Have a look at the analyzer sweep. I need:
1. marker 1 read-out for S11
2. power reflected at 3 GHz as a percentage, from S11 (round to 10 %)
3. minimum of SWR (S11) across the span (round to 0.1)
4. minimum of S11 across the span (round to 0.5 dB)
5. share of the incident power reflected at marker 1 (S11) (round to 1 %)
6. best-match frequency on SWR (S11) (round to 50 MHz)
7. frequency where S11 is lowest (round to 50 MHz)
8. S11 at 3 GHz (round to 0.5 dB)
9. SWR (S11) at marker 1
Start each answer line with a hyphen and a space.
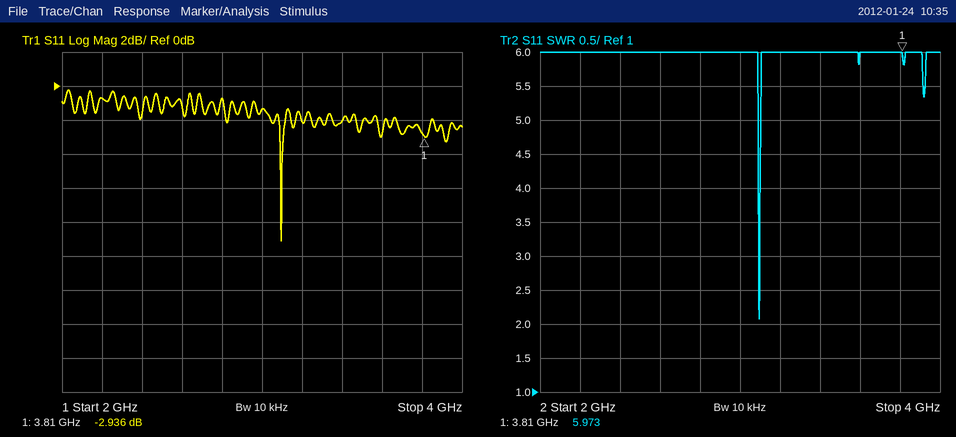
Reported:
- -2.936 dB
- 70 %
- 2.1
- -9.0 dB
- 51 %
- 3.10 GHz
- 3.10 GHz
- -1.5 dB
- 5.973
